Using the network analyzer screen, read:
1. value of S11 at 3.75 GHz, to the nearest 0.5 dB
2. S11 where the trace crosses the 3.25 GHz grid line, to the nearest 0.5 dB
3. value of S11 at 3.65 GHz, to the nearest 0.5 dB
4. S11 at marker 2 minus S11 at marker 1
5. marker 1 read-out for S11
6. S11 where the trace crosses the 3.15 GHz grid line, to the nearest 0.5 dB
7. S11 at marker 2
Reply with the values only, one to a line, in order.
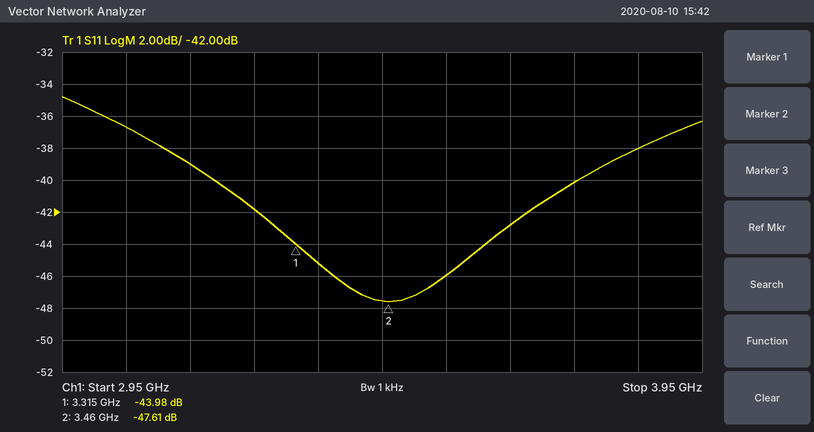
-40.0 dB
-42.0 dB
-43.0 dB
-3.63 dB
-43.98 dB
-39.0 dB
-47.61 dB
